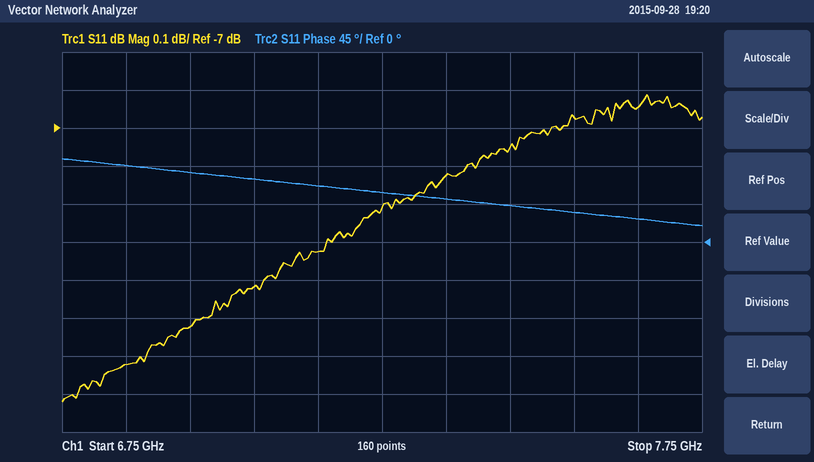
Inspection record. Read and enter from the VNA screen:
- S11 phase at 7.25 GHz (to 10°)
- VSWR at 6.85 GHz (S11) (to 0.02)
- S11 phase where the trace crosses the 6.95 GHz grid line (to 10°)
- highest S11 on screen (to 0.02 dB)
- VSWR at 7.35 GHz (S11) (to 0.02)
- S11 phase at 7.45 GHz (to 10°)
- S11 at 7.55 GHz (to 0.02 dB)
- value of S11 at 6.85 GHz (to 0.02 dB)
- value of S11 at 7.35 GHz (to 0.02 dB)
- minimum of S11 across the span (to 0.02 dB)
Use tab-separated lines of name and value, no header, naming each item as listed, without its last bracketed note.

S11 phase at 7.25 GHz	60°
VSWR at 6.85 GHz (S11)	2.42
S11 phase where the trace crosses the 6.95 GHz grid line	80°
highest S11 on screen	-6.92 dB
VSWR at 7.35 GHz (S11)	2.58
S11 phase at 7.45 GHz	40°
S11 at 7.55 GHz	-6.98 dB
value of S11 at 6.85 GHz	-7.62 dB
value of S11 at 7.35 GHz	-7.12 dB
minimum of S11 across the span	-7.72 dB
